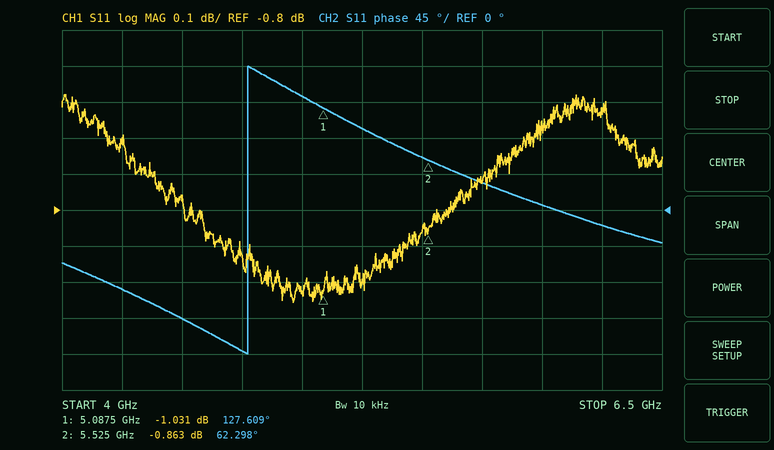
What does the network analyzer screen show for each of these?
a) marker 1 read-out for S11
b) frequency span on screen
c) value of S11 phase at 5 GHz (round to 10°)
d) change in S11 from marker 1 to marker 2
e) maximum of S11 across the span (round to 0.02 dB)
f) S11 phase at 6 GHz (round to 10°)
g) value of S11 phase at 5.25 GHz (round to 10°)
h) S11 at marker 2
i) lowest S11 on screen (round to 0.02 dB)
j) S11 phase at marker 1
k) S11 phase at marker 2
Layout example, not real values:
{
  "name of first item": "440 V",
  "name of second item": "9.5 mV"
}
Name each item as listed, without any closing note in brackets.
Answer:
{
  "marker 1 read-out for S11": "-1.031 dB",
  "frequency span on screen": "2.5 GHz",
  "value of S11 phase at 5 GHz": "140°",
  "change in S11 from marker 1 to marker 2": "0.168 dB",
  "maximum of S11 across the span": "-0.48 dB",
  "S11 phase at 6 GHz": "10°",
  "value of S11 phase at 5.25 GHz": "100°",
  "S11 at marker 2": "-0.863 dB",
  "lowest S11 on screen": "-1.06 dB",
  "S11 phase at marker 1": "127.609°",
  "S11 phase at marker 2": "62.298°"
}
